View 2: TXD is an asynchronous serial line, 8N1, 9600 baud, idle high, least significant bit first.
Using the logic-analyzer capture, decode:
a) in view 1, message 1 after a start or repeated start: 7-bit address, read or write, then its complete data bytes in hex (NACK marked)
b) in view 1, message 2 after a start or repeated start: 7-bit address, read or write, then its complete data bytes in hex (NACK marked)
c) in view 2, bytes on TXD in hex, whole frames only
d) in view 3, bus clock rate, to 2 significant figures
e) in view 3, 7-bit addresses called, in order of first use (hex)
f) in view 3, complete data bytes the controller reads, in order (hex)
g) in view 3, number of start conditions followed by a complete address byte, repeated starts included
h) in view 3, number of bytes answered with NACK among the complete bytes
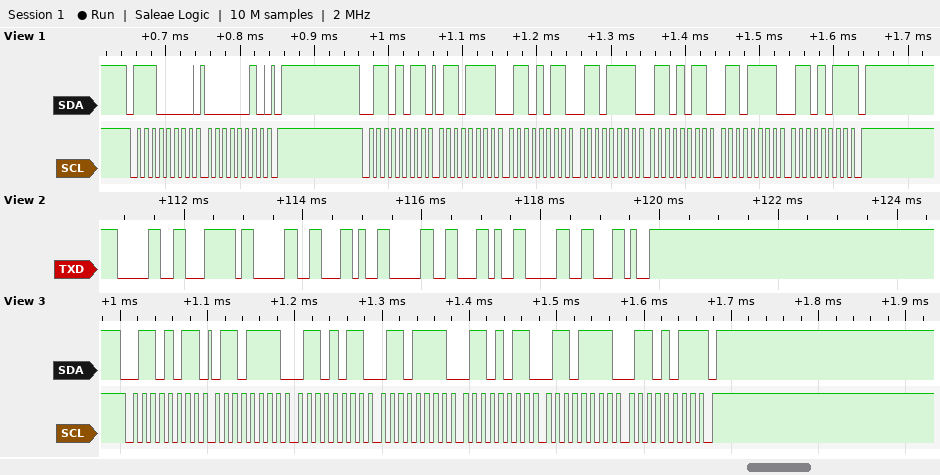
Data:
0x70 write: 02
0x35 read: 6F 6B 6F 6B 6F 6B NACK
30 7C 30 2C 30 2C 30 2C
100 kHz
0x35
6F 6B 6F 6B 6F 6B
1
1
